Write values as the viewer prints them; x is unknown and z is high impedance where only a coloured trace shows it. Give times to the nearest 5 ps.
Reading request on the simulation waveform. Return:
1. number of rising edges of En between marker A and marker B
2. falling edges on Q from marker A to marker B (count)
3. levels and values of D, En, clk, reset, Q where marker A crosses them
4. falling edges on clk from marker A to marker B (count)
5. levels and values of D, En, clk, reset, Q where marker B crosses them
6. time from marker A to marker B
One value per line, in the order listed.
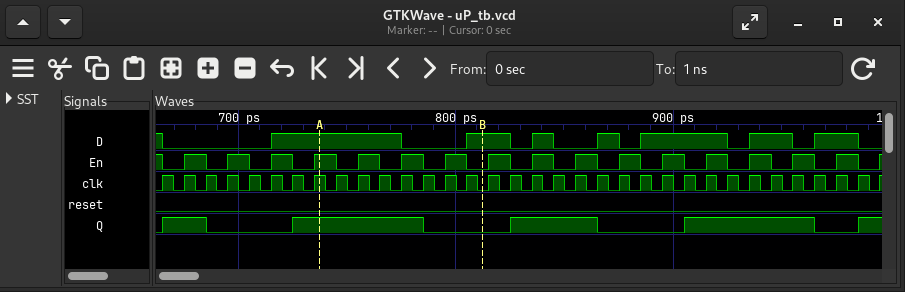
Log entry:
3
1
D=1, En=1, clk=1, reset=0, Q=1
8
D=1, En=0, clk=0, reset=0, Q=0
75 ps
